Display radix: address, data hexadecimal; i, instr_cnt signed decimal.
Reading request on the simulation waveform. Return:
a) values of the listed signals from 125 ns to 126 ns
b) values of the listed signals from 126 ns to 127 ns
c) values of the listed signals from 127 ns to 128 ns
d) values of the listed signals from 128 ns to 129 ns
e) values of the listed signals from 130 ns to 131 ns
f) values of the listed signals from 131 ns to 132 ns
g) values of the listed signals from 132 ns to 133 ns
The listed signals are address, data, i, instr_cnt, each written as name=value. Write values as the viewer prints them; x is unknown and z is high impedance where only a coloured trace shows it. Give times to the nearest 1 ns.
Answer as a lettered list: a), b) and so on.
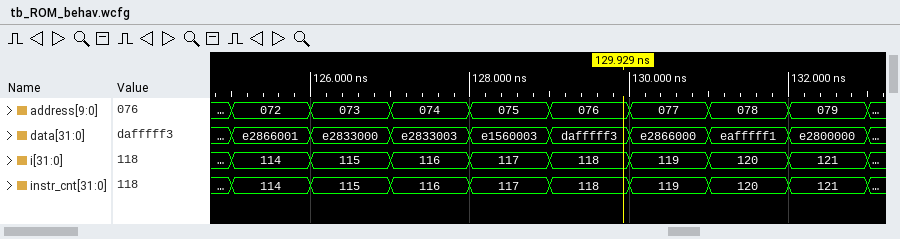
a) address=072, data=e2866001, i=114, instr_cnt=114
b) address=073, data=e2833000, i=115, instr_cnt=115
c) address=074, data=e2833003, i=116, instr_cnt=116
d) address=075, data=e1560003, i=117, instr_cnt=117
e) address=077, data=e2866000, i=119, instr_cnt=119
f) address=078, data=eafffff1, i=120, instr_cnt=120
g) address=079, data=e2800000, i=121, instr_cnt=121
